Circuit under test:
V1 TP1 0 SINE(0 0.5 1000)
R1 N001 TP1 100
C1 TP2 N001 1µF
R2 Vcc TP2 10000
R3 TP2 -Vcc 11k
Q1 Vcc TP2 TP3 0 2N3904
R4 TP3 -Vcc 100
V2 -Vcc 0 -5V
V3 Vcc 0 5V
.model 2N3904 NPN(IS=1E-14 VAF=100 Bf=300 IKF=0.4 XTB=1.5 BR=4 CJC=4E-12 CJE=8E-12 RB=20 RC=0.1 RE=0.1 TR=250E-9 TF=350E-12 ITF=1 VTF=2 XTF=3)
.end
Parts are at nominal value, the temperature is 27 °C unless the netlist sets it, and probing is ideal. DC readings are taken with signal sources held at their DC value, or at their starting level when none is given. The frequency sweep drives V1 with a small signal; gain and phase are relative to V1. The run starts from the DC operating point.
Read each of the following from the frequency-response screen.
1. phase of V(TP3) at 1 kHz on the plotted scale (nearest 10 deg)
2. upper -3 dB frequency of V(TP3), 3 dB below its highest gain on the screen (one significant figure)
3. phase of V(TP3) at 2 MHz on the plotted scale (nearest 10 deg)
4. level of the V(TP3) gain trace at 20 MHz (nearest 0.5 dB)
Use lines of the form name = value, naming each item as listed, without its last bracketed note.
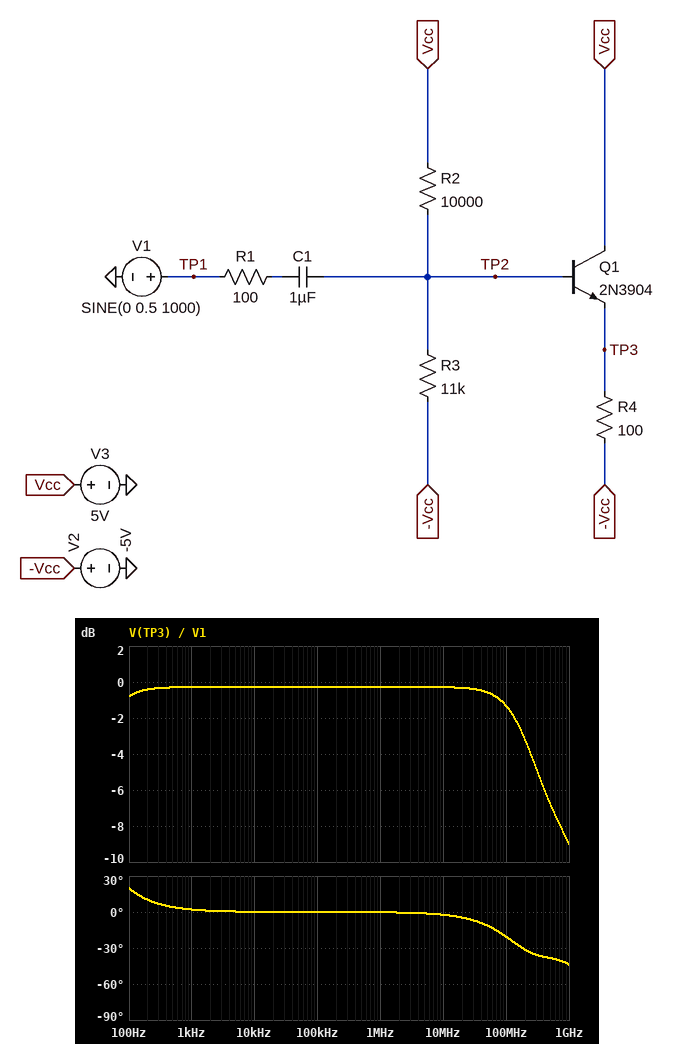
phase of V(TP3) at 1 kHz on the plotted scale = 0 deg
upper -3 dB frequency of V(TP3), 3 dB below its highest gain on the screen = 200 MHz
phase of V(TP3) at 2 MHz on the plotted scale = 0 deg
level of the V(TP3) gain trace at 20 MHz = -0.5 dB
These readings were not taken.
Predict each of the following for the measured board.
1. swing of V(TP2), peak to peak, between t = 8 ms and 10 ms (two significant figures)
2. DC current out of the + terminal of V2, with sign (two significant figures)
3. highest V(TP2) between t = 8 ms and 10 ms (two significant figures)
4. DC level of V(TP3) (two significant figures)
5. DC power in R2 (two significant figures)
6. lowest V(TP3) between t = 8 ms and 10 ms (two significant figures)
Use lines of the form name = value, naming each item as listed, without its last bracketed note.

swing of V(TP2), peak to peak, between t = 8 ms and 10 ms = 980 mV
DC current out of the + terminal of V2, with sign = -38 mA
highest V(TP2) between t = 8 ms and 10 ms = 41 mV
DC level of V(TP3) = -1.2 V
DC power in R2 = 3.0 mW
lowest V(TP3) between t = 8 ms and 10 ms = -1.7 V
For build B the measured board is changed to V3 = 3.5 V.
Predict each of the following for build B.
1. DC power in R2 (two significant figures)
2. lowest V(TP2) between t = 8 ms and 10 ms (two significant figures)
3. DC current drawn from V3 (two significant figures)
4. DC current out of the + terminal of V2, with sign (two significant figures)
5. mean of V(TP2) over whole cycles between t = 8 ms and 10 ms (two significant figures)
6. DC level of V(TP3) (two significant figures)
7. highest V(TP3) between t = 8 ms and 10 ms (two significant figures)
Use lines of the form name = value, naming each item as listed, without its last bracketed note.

DC power in R2 = 2.1 mW
lowest V(TP2) between t = 8 ms and 10 ms = -1.6 V
DC current drawn from V3 = 32 mA
DC current out of the + terminal of V2, with sign = -32 mA
mean of V(TP2) over whole cycles between t = 8 ms and 10 ms = -1.1 V
DC level of V(TP3) = -1.9 V
highest V(TP3) between t = 8 ms and 10 ms = -1.4 V
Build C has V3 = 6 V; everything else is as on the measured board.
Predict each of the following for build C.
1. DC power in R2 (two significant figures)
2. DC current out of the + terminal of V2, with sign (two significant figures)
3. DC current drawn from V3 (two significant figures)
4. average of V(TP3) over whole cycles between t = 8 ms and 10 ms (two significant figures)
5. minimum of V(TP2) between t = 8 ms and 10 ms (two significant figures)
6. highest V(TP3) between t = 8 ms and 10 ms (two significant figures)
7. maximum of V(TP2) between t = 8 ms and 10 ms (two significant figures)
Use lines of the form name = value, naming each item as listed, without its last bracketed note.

DC power in R2 = 3.6 mW
DC current out of the + terminal of V2, with sign = -43 mA
DC current drawn from V3 = 43 mA
average of V(TP3) over whole cycles between t = 8 ms and 10 ms = -770 mV
minimum of V(TP2) between t = 8 ms and 10 ms = -490 mV
highest V(TP3) between t = 8 ms and 10 ms = -280 mV
maximum of V(TP2) between t = 8 ms and 10 ms = 480 mV
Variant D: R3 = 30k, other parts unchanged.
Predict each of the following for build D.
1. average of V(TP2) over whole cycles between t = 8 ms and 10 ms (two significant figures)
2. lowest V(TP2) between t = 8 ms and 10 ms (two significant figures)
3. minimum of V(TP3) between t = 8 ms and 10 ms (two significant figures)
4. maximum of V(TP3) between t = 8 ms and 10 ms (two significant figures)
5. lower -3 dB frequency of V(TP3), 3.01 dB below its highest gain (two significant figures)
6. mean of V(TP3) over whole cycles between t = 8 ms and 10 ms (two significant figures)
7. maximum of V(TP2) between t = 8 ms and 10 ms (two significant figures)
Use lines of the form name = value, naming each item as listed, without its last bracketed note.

average of V(TP2) over whole cycles between t = 8 ms and 10 ms = 1.1 V
lowest V(TP2) between t = 8 ms and 10 ms = 570 mV
minimum of V(TP3) between t = 8 ms and 10 ms = -190 mV
maximum of V(TP3) between t = 8 ms and 10 ms = 780 mV
lower -3 dB frequency of V(TP3), 3.01 dB below its highest gain = 27 Hz
mean of V(TP3) over whole cycles between t = 8 ms and 10 ms = 300 mV
maximum of V(TP2) between t = 8 ms and 10 ms = 1.6 V
